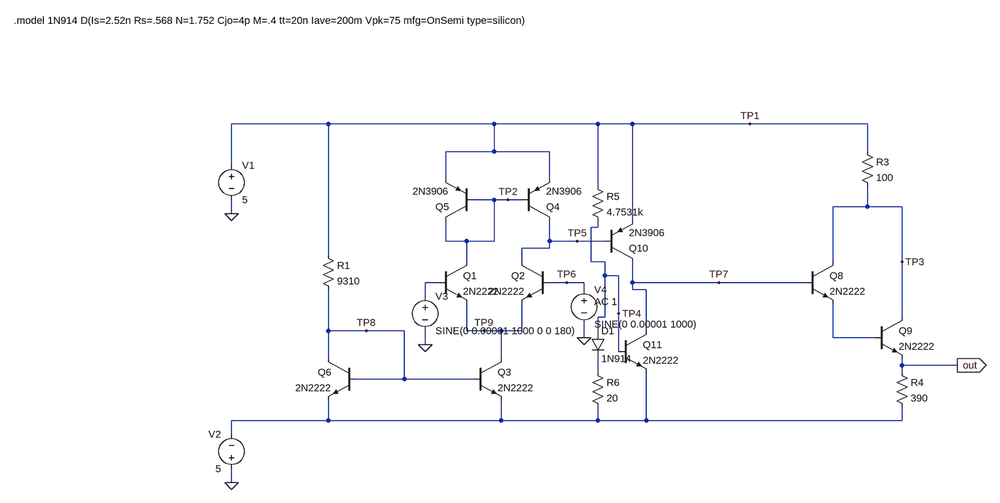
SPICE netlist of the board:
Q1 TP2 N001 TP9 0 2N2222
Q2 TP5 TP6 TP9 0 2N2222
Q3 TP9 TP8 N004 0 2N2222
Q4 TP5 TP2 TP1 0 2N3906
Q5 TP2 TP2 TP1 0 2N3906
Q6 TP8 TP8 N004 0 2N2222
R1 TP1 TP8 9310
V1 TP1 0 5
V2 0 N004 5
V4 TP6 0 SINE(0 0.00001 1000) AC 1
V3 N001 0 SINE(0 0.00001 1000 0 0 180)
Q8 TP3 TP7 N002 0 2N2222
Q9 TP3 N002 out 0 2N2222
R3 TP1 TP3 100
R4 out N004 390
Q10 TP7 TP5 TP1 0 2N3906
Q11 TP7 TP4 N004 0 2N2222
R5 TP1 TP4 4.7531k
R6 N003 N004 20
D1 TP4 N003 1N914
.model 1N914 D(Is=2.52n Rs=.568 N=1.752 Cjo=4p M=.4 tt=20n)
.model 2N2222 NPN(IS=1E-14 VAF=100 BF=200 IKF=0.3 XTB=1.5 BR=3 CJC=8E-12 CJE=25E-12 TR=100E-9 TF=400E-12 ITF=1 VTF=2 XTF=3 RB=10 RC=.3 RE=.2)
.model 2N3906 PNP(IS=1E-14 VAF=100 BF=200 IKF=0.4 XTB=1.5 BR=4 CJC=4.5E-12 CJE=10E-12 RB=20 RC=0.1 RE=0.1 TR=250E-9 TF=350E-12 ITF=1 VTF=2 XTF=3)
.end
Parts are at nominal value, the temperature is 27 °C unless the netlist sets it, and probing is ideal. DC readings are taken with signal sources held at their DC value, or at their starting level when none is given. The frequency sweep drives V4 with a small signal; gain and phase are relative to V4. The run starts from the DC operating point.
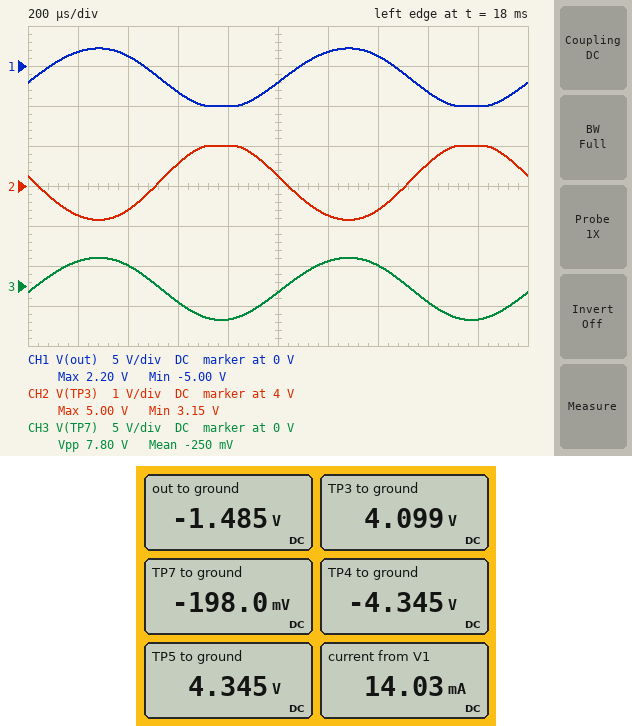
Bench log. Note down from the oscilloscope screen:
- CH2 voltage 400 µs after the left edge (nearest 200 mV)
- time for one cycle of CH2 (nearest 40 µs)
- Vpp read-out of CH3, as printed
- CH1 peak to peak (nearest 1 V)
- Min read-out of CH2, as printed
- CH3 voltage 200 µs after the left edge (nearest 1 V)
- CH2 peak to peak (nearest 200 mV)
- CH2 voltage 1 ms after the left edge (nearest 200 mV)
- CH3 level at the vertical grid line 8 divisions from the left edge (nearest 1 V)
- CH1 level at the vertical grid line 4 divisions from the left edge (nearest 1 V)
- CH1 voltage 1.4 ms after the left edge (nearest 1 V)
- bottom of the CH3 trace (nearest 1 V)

3.4 V
1.00 ms
7.80 V
7 V
3.15 V
3 V
1.8 V
4.2 V
-2 V
-5 V
1 V
-4 V
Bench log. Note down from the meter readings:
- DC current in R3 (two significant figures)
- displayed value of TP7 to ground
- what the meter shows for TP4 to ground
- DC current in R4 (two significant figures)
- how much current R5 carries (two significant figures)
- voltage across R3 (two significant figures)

9.0 mA
-198.0 mV
-4.345 V
9.0 mA
2.0 mA
900 mV
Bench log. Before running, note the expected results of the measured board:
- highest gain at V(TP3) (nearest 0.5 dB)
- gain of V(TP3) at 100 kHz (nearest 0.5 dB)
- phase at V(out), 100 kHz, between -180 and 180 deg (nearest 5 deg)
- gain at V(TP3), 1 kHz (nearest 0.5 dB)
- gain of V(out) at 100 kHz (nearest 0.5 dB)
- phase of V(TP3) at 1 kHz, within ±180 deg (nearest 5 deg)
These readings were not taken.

94.0 dB
70.0 dB
-85 deg
94.0 dB
82.0 dB
170 deg
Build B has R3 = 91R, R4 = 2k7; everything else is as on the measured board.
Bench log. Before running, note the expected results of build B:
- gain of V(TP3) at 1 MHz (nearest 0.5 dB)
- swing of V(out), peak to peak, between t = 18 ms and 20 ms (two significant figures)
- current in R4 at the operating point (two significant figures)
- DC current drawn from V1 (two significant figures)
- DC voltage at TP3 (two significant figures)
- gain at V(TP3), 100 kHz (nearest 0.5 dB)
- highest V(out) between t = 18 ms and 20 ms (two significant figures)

32.5 dB
7.3 V
1.3 mA
6.4 mA
4.9 V
52.5 dB
2.3 V
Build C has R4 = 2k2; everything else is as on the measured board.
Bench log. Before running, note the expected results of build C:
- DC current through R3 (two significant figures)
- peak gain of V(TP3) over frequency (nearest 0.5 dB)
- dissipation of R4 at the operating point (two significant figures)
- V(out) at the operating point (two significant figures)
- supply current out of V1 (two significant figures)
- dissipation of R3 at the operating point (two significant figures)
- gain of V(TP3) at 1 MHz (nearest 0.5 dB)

1.6 mA
79.0 dB
5.9 mW
-1.4 V
6.7 mA
270 µW
35.0 dB
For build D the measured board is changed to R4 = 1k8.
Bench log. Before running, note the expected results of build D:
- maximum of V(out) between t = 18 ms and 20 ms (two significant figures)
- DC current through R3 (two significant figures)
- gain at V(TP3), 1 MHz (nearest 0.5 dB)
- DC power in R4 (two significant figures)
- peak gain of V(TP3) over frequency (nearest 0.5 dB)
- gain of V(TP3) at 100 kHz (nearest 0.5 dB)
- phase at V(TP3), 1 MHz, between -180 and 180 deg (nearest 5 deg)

2.3 V
2.0 mA
36.5 dB
7.2 mW
80.5 dB
56.5 dB
80 deg
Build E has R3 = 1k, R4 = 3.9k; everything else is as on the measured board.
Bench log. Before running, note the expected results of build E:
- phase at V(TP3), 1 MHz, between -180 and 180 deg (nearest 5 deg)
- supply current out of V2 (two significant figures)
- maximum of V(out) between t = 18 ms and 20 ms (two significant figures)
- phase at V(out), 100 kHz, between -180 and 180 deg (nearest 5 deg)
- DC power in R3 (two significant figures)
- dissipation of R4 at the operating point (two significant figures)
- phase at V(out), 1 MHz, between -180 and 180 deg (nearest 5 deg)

70 deg
6.0 mA
2.3 V
-90 deg
870 µW
3.4 mW
-100 deg
